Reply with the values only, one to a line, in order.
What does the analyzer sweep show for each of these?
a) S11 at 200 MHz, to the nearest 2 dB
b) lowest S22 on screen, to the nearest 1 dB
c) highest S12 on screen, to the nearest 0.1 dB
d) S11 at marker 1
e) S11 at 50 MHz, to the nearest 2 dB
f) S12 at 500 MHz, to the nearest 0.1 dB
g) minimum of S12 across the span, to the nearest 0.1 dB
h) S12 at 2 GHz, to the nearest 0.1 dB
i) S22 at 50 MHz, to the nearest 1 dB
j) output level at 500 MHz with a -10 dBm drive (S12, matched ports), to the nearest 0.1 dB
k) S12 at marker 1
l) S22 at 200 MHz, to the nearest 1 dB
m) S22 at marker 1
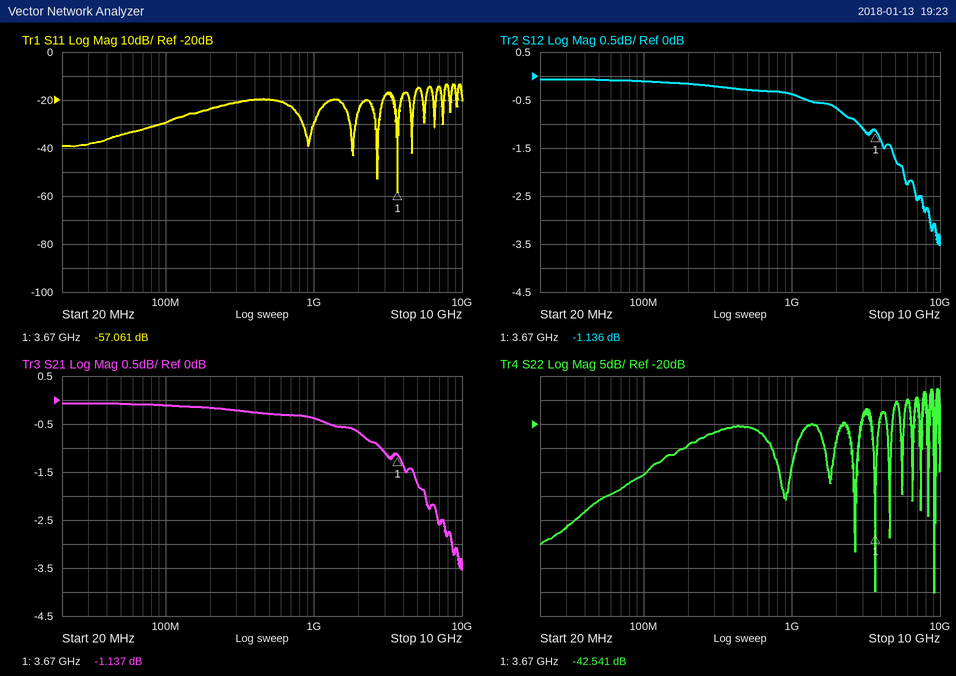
-24 dB
-55 dB
-0.1 dB
-57.061 dB
-34 dB
-0.3 dB
-3.5 dB
-0.7 dB
-36 dB
-10.3 dBm
-1.136 dB
-24 dB
-42.541 dB
